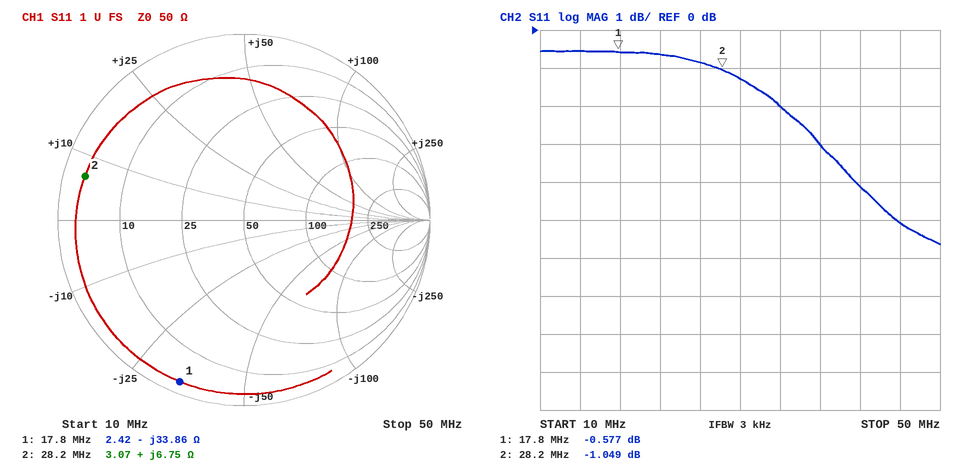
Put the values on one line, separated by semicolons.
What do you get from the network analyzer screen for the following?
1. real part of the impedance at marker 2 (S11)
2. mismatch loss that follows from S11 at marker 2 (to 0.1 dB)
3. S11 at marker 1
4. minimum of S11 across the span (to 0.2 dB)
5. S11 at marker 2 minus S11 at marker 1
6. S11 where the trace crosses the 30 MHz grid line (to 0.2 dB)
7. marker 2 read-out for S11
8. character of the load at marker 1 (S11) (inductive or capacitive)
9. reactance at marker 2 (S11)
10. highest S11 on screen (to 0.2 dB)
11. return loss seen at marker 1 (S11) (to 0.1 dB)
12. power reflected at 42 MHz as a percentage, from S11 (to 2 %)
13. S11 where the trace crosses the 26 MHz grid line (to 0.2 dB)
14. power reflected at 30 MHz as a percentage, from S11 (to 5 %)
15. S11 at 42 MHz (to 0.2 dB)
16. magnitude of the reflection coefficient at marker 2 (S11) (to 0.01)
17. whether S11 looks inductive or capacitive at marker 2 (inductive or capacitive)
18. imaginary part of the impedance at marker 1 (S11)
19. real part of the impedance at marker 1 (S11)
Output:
3.07 Ω; 6.7 dB; -0.577 dB; -5.6 dB; -0.472 dB; -1.2 dB; -1.049 dB; capacitive; +6.75 Ω; -0.6 dB; 0.6 dB; 38 %; -0.8 dB; 75 %; -4.2 dB; 0.89; inductive; -33.86 Ω; 2.42 Ω
